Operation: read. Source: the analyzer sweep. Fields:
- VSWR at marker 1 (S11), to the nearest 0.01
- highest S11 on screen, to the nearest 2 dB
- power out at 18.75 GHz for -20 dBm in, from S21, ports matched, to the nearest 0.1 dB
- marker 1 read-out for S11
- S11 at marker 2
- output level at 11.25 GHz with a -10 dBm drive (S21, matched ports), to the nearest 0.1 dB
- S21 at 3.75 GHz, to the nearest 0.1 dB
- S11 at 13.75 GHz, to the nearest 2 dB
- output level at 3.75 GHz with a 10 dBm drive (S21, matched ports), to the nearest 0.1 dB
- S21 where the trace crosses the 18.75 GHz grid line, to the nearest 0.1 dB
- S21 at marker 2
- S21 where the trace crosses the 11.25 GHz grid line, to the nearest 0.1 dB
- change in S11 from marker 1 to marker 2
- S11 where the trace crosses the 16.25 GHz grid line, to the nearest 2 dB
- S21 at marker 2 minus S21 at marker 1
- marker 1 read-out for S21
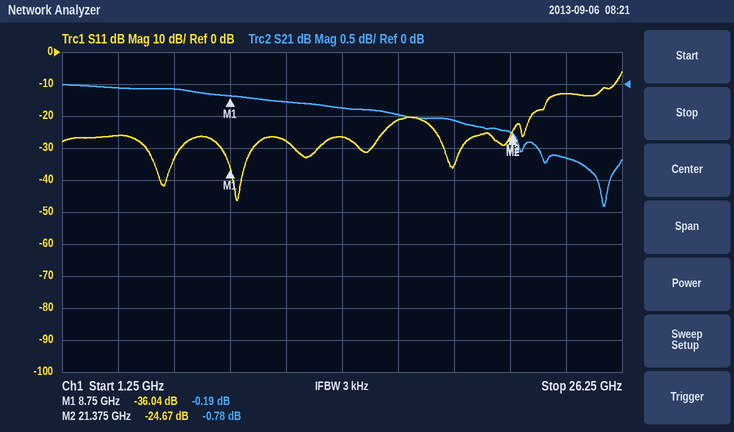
1.03
-6 dB
-20.6 dBm
-36.04 dB
-24.67 dB
-10.3 dBm
-0.1 dB
-26 dB
9.9 dBm
-0.6 dB
-0.78 dB
-0.3 dB
11.37 dB
-22 dB
-0.59 dB
-0.19 dB
